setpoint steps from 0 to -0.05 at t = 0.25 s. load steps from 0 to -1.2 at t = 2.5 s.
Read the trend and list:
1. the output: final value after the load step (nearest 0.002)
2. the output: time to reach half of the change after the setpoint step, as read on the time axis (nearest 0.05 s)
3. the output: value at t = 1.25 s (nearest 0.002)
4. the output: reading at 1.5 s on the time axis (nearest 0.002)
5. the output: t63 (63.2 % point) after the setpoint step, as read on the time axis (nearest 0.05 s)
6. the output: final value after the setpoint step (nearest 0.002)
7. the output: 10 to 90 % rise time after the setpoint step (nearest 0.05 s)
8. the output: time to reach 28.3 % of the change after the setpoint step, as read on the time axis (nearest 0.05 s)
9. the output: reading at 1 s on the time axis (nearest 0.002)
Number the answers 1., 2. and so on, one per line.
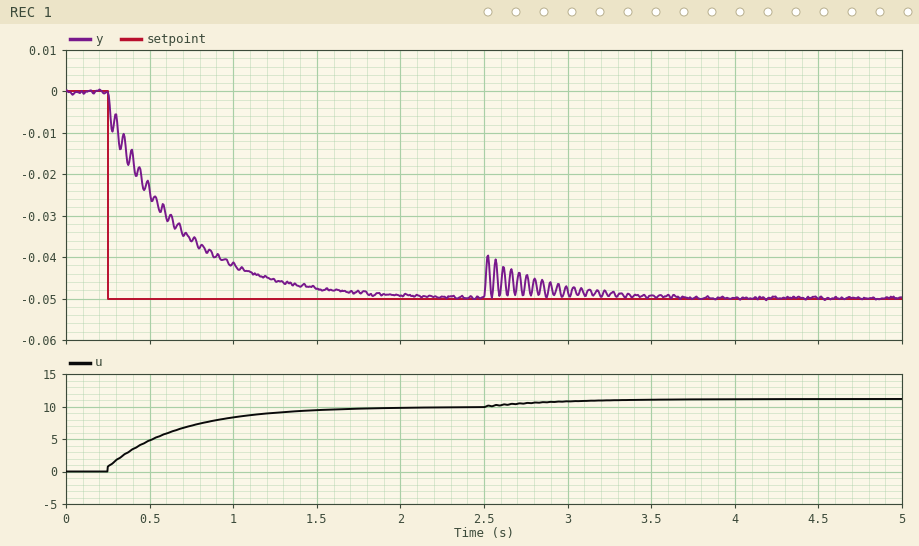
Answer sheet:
1. -0.050
2. 0.50 s
3. -0.046
4. -0.048
5. 0.65 s
6. -0.050
7. 0.95 s
8. 0.35 s
9. -0.042
